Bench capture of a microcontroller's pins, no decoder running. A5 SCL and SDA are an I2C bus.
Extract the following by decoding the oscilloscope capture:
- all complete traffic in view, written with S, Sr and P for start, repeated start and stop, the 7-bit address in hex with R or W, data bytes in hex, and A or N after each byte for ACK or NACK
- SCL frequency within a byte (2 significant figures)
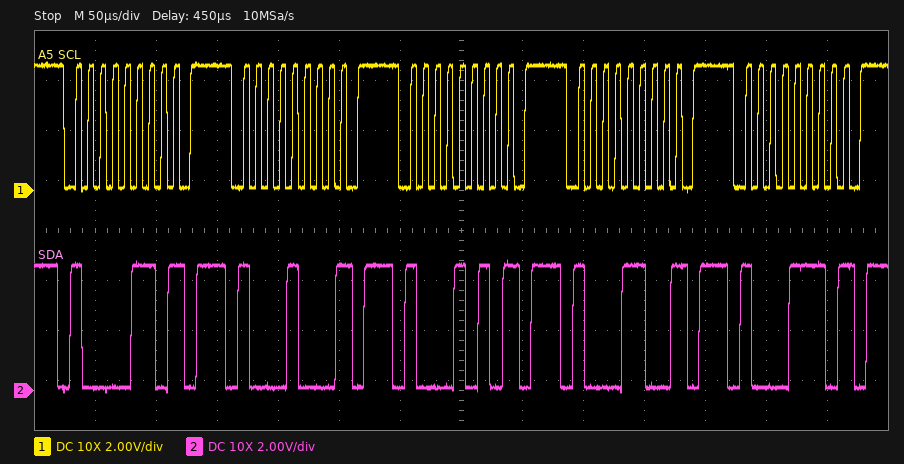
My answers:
S 43W N P S 44W N P S 45W N P S 46W N P S 47W N P
100 kHz
